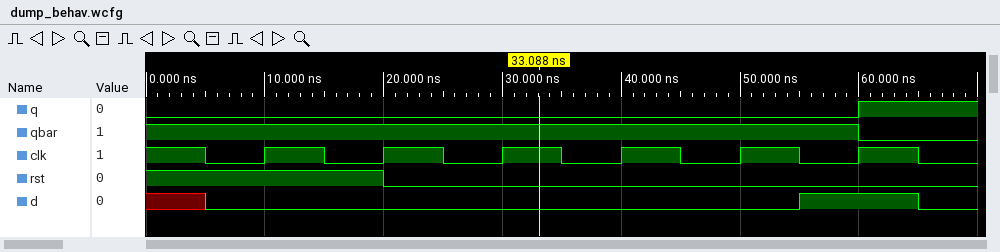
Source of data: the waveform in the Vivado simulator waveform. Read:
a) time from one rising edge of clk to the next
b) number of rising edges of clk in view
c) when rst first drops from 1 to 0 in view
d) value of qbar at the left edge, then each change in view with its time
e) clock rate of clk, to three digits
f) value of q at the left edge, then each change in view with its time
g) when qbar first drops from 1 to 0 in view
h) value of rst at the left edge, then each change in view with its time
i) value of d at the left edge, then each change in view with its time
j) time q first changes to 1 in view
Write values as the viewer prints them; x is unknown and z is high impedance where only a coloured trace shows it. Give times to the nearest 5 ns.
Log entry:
10 ns
6
20 ns
1, 0 at 60 ns
100 MHz
0, 1 at 60 ns
60 ns
1, 0 at 20 ns
x, 0 at 5 ns, 1 at 55 ns, 0 at 65 ns
60 ns
